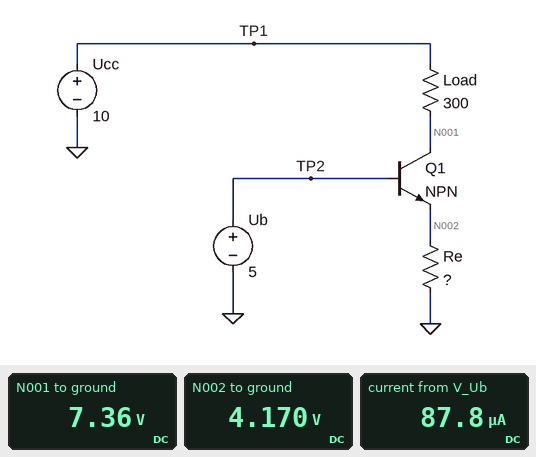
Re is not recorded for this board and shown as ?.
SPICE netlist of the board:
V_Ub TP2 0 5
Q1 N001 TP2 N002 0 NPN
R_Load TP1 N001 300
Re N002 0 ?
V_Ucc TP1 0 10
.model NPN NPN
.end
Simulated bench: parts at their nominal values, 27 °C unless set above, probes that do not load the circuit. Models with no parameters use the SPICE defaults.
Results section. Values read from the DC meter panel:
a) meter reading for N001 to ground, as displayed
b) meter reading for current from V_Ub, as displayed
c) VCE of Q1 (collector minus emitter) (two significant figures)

7.36 V
87.8 µA
3.2 V
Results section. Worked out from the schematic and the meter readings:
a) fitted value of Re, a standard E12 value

470 Ω
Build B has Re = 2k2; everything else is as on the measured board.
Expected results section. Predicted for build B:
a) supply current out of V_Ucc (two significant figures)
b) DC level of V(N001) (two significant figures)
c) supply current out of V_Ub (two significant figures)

1.9 mA
9.4 V
19 µA
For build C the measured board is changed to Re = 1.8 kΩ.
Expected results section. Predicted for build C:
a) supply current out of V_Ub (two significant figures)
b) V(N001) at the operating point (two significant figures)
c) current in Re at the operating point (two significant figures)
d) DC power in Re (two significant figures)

23 µA
9.3 V
2.3 mA
9.8 mW
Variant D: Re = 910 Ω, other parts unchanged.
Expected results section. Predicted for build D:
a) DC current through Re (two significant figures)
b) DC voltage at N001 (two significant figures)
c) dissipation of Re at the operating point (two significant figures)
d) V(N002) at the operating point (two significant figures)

4.6 mA
8.6 V
19 mW
4.2 V
